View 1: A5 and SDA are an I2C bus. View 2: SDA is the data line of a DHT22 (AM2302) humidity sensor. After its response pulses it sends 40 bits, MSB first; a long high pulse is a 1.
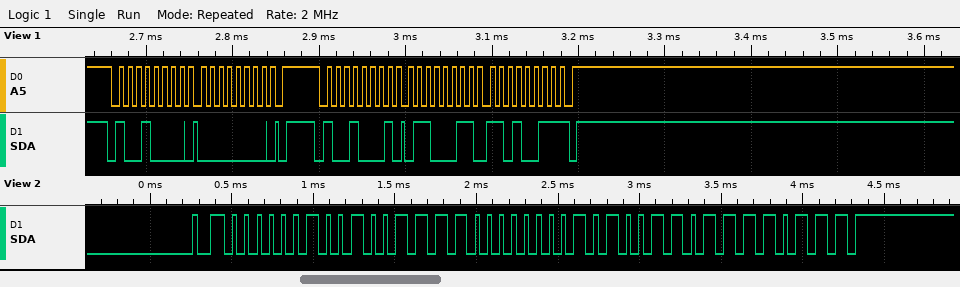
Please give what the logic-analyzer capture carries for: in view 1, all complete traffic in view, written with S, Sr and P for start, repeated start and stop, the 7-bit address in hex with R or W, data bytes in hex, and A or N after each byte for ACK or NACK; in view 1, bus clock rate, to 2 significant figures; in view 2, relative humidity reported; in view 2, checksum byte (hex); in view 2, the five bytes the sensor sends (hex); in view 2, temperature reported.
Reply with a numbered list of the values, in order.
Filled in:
1. S 48W A 00 A P S 48R A 63 A D3 N P
2. 100 kHz
3. 59.1 %
4. 0xF7
5. 02 4F 00 A6 F7
6. 16.6 °C
